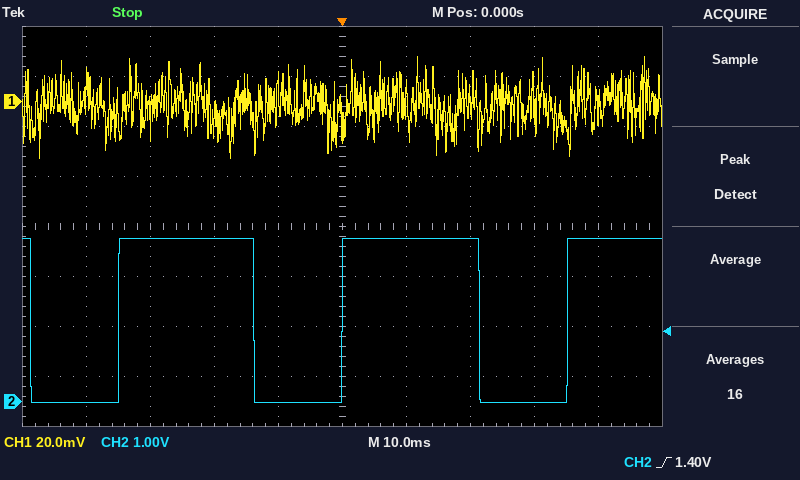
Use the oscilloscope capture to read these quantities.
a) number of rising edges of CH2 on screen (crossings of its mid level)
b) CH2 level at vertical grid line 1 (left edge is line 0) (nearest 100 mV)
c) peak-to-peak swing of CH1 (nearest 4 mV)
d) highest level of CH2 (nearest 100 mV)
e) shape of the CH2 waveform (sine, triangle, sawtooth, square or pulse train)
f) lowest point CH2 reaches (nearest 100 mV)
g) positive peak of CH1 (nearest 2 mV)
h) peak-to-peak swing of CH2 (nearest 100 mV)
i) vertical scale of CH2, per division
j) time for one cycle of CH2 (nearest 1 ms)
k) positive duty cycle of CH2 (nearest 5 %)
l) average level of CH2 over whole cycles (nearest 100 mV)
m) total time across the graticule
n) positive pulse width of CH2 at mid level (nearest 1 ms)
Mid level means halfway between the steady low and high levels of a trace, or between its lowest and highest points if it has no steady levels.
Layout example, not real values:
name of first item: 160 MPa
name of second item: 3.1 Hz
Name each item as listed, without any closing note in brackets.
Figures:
number of rising edges of CH2 on screen: 3
CH2 level at vertical grid line 1 (left edge is line 0): 0.0 V
peak-to-peak swing of CH1: 40 mV
highest level of CH2: 3.3 V
shape of the CH2 waveform: pulse train
lowest point CH2 reaches: 0.0 V
positive peak of CH1: 18 mV
peak-to-peak swing of CH2: 3.3 V
vertical scale of CH2, per division: 1 V
time for one cycle of CH2: 35 ms
positive duty cycle of CH2: 60 %
average level of CH2 over whole cycles: 2.0 V
total time across the graticule: 100 ms
positive pulse width of CH2 at mid level: 21 ms
